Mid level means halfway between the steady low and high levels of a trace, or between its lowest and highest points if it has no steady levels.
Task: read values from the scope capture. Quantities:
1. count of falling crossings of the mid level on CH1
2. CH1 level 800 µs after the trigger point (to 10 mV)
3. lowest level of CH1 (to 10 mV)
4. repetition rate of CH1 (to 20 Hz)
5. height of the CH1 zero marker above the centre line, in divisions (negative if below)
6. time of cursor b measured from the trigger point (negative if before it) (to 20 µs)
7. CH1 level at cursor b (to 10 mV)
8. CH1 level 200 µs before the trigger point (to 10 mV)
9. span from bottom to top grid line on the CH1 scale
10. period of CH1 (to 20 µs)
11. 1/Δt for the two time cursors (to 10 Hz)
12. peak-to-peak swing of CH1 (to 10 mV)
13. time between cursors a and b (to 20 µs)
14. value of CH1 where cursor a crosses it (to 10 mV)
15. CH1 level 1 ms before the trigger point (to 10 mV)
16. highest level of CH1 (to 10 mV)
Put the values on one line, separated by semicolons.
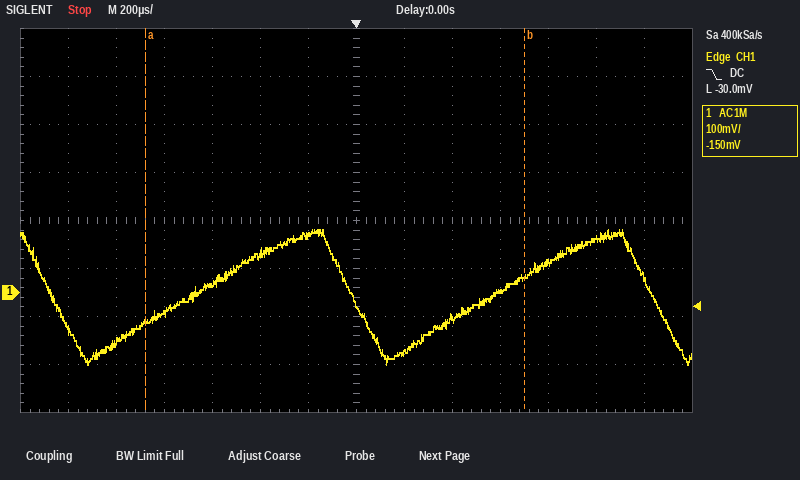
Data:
3; 60 mV; -150 mV; 800 Hz; -1.5 div; +700 µs; 30 mV; 120 mV; 800 mV; 1.26 ms; 630 Hz; 280 mV; 1.58 ms; -60 mV; -100 mV; 130 mV
